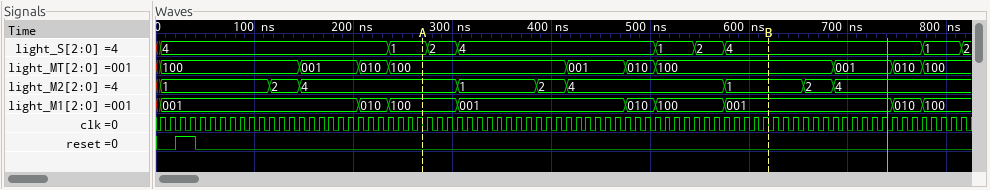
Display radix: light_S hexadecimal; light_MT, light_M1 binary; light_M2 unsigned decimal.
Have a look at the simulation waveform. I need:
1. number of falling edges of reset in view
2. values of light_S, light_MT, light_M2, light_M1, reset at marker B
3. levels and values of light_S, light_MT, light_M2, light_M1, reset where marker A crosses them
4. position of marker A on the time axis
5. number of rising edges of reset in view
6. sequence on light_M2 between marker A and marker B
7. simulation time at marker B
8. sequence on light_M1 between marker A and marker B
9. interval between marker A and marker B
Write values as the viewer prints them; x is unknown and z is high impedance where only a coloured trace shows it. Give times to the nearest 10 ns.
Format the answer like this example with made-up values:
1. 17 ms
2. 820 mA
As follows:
1. 1
2. light_S=4, light_MT=100, light_M2=1, light_M1=001, reset=0
3. light_S=1, light_MT=100, light_M2=4, light_M1=100, reset=0
4. 270 ns
5. 1
6. 4, 1, 2, 4, 1
7. 620 ns
8. 100, 001, 010, 100, 001
9. 350 ns
